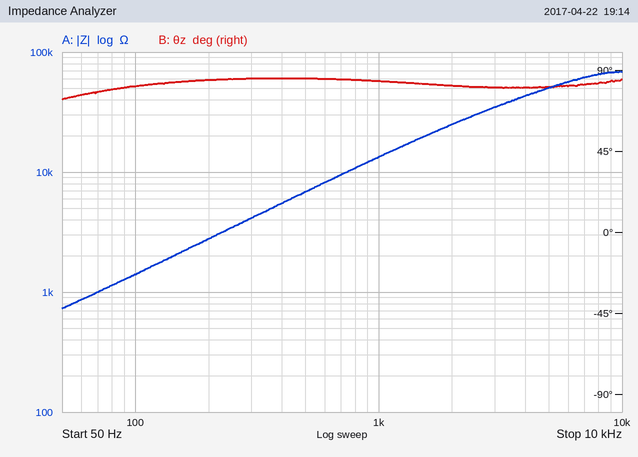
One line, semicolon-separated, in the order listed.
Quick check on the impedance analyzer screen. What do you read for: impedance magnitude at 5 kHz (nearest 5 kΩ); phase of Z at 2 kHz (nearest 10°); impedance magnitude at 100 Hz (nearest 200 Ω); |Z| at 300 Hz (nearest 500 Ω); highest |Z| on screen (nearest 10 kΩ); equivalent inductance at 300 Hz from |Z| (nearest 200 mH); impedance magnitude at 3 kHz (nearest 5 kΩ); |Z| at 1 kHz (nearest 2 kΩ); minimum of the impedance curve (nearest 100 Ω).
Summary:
50 kΩ; 80°; 1.4 kΩ; 4.0 kΩ; 70 kΩ; 2.2 H; 35 kΩ; 14 kΩ; 700 Ω
